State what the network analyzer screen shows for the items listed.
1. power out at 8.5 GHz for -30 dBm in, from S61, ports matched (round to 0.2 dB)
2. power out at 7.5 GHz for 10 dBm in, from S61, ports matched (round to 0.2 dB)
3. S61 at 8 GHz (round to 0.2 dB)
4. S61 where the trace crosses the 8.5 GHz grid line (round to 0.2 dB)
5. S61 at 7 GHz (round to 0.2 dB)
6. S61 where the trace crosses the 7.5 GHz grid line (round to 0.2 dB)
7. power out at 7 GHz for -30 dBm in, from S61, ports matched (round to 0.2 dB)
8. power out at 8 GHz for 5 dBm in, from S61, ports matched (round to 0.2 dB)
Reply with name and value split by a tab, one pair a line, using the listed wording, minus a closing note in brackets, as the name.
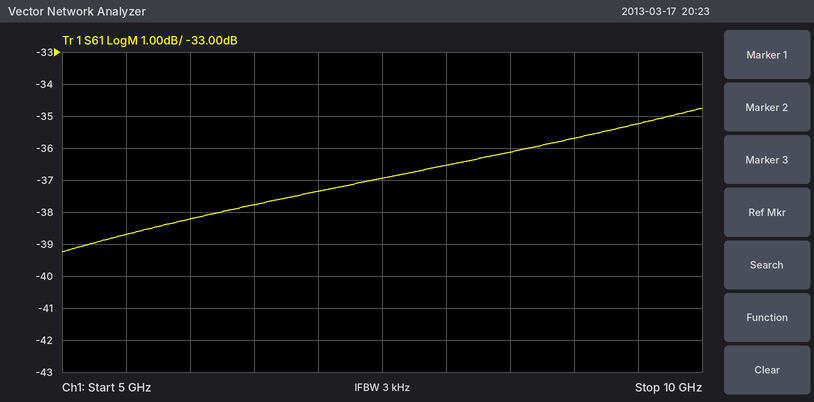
power out at 8.5 GHz for -30 dBm in, from S61, ports matched	-66.2 dBm
power out at 7.5 GHz for 10 dBm in, from S61, ports matched	-27.0 dBm
S61 at 8 GHz	-36.6 dB
S61 where the trace crosses the 8.5 GHz grid line	-36.2 dB
S61 at 7 GHz	-37.4 dB
S61 where the trace crosses the 7.5 GHz grid line	-37.0 dB
power out at 7 GHz for -30 dBm in, from S61, ports matched	-67.4 dBm
power out at 8 GHz for 5 dBm in, from S61, ports matched	-31.6 dBm
